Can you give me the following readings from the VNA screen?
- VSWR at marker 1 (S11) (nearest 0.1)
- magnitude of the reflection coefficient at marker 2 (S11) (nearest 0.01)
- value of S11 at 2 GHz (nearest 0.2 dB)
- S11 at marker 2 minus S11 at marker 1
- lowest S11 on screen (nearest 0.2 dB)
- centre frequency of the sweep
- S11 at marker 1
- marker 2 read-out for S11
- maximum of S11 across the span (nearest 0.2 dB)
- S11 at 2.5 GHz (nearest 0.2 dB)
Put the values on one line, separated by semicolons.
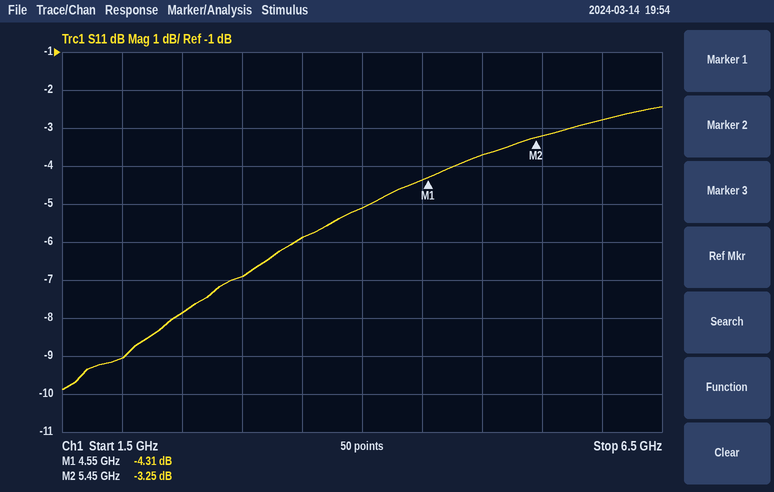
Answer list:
4.1; 0.69; -9.0 dB; 1.06 dB; -9.8 dB; 4 GHz; -4.31 dB; -3.25 dB; -2.4 dB; -7.8 dB
